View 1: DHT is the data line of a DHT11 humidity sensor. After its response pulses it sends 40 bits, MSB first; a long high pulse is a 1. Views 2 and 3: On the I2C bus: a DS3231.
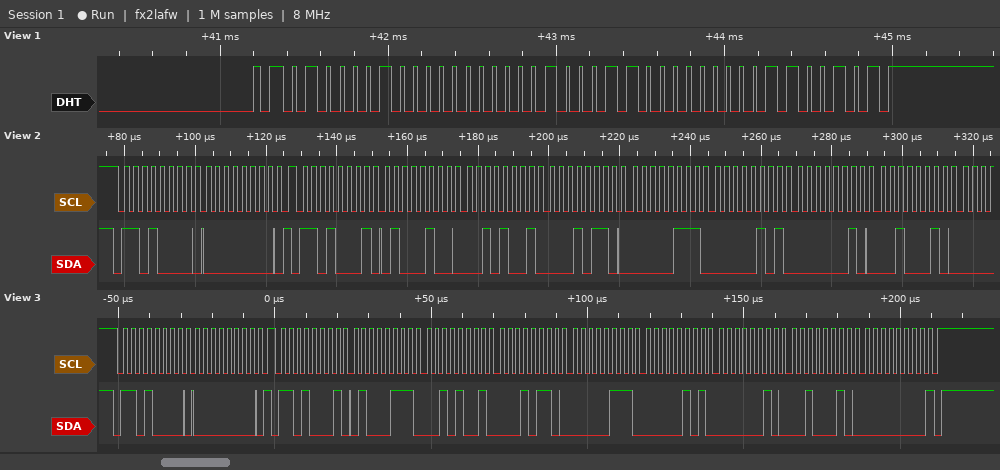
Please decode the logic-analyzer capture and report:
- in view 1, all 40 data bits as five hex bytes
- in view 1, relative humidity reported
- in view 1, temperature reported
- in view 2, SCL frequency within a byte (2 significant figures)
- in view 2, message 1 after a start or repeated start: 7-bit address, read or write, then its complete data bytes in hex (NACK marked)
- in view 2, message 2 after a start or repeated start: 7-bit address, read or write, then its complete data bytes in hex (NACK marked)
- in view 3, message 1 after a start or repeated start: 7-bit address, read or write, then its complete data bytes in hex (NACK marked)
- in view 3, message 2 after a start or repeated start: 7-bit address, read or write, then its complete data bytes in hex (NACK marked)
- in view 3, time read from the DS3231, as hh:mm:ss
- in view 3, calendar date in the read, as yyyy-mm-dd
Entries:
42 00 23 00 65
66 %
35.0 °C
400 kHz
0x68 write: 00
0x68 read: 44 29 16 07 05 02 22
0x68 write: 00
0x68 read: 47 29 16 07 05 02 22 00 NACK
16:29:47
2022-02-05
